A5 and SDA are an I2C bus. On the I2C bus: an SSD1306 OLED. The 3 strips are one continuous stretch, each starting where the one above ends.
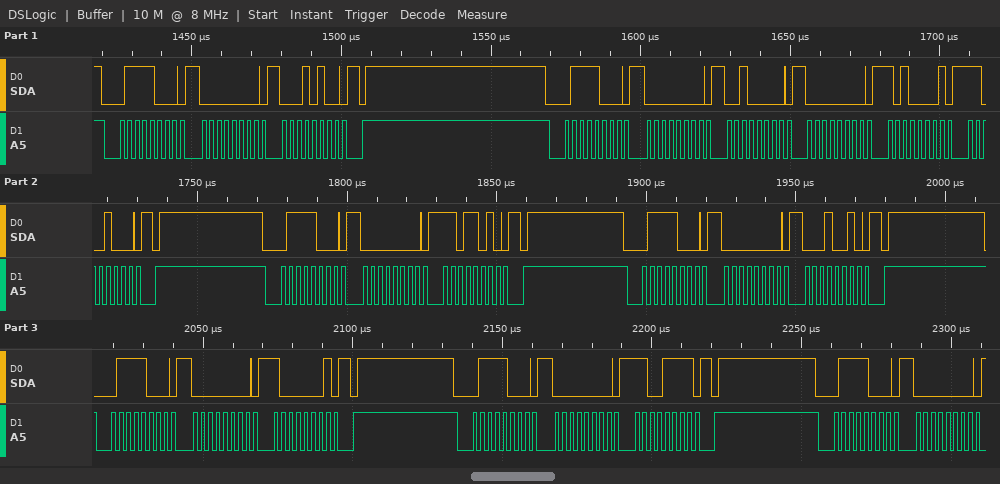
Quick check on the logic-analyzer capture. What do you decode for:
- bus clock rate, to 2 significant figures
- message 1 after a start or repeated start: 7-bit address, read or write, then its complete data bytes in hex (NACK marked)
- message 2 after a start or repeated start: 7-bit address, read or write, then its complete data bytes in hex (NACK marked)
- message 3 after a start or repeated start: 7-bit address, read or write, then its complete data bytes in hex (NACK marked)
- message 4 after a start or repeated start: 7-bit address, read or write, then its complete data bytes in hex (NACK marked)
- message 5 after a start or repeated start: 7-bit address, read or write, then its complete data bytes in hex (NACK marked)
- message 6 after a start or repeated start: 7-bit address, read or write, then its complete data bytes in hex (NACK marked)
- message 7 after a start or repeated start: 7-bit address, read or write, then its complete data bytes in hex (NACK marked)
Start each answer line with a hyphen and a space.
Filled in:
- 400 kHz
- 0x3C write: 00 14
- 0x3C write: 00 20 00 A1 C8
- 0x3C write: 00 DA
- 0x3C write: 00 12
- 0x3C write: 00 81
- 0x3C write: 00 CF
- 0x3C write: 00
